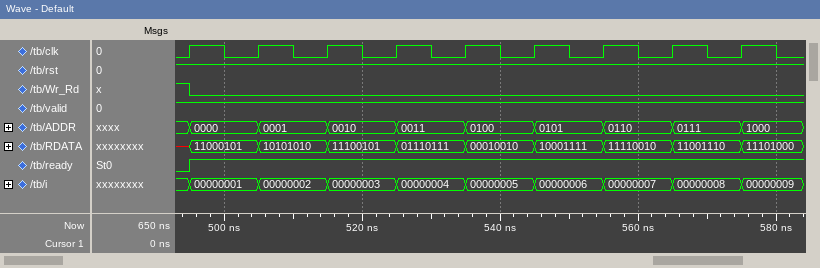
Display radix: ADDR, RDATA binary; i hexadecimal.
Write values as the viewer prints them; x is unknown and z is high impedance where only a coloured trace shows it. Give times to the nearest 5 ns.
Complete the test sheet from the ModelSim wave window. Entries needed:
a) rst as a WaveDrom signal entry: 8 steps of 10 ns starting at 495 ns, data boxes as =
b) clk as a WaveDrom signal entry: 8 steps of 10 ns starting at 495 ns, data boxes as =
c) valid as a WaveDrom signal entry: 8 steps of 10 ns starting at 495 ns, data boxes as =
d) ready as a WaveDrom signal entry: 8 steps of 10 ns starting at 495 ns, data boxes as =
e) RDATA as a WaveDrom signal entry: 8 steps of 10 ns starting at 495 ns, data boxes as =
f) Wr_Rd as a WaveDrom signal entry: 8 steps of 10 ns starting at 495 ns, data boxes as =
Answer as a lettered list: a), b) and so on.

a) {name: 'rst', wave: '1.......'}
b) {name: 'clk', wave: 'p.......'}
c) {name: 'valid', wave: '1.......'}
d) {name: 'ready', wave: '1.......'}
e) {name: 'RDATA', wave: '========', data: '11000101 10101010 11100101 01110111 00010010 10001111 11110010 11001110'}
f) {name: 'Wr_Rd', wave: '0.......'}
